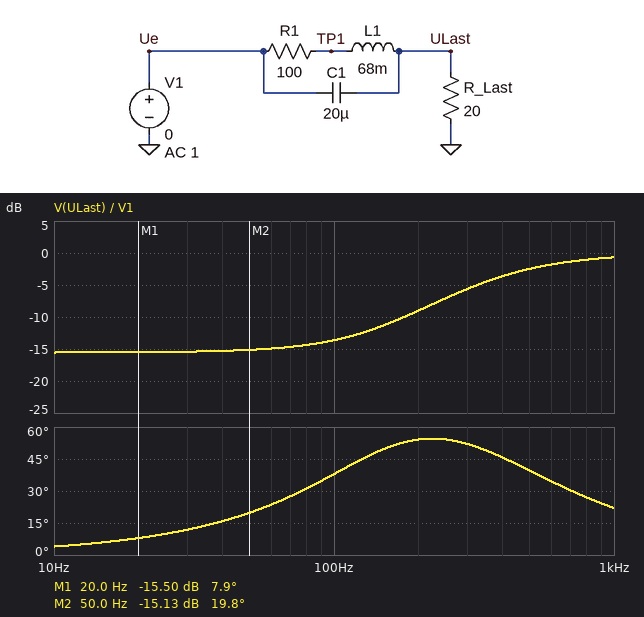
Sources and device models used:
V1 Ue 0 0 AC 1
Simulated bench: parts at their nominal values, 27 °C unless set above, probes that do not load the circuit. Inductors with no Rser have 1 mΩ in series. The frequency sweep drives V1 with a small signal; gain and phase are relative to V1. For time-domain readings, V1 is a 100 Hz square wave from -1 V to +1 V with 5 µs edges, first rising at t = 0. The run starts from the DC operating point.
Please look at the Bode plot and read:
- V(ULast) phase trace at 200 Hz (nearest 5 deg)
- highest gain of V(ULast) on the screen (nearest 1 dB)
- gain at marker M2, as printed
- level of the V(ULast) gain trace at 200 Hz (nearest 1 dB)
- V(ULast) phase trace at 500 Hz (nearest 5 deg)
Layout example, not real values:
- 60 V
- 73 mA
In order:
- 55 deg
- -1 dB
- -15.13 dB
- -9 dB
- 40 deg
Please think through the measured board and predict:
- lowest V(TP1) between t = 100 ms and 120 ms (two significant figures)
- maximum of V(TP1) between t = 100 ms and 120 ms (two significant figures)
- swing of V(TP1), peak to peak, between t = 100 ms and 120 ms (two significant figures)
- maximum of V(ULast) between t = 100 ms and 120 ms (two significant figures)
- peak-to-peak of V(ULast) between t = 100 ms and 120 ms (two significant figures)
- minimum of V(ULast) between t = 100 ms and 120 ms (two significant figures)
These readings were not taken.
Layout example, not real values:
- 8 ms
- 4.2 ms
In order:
- -1.8 V
- 1.8 V
- 3.7 V
- 1.8 V
- 3.6 V
- -1.8 V
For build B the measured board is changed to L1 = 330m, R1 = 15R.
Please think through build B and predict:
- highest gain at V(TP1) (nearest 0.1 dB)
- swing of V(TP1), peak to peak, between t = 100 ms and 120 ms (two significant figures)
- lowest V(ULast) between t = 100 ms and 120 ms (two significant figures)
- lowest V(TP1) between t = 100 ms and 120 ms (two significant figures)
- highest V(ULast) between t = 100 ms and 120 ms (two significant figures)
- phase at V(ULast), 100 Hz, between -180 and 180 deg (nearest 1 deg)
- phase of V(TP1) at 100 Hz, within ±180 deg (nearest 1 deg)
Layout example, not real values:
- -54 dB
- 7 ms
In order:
- 0.1 dB
- 2.2 V
- -1.9 V
- -1.1 V
- 1.9 V
- 79 deg
- 4 deg
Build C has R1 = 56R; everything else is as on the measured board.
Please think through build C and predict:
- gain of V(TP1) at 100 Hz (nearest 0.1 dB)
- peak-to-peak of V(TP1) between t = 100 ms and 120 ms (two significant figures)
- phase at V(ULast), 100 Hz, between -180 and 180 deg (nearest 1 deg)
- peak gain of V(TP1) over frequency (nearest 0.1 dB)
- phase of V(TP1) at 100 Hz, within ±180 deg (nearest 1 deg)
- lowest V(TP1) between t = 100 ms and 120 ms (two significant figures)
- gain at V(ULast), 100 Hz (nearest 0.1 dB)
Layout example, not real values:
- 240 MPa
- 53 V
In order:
- -3.5 dB
- 3.5 V
- 16 deg
- 0.9 dB
- 40 deg
- -1.7 V
- -14.2 dB
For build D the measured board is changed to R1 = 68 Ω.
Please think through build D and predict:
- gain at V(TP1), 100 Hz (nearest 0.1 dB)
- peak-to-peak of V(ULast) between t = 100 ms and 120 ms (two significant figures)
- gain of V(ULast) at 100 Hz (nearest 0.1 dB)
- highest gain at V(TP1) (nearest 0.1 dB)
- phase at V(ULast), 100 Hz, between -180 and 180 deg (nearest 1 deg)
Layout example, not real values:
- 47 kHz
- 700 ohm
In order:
- -4.2 dB
- 3.5 V
- -14.0 dB
- 1.0 dB
- 24 deg
